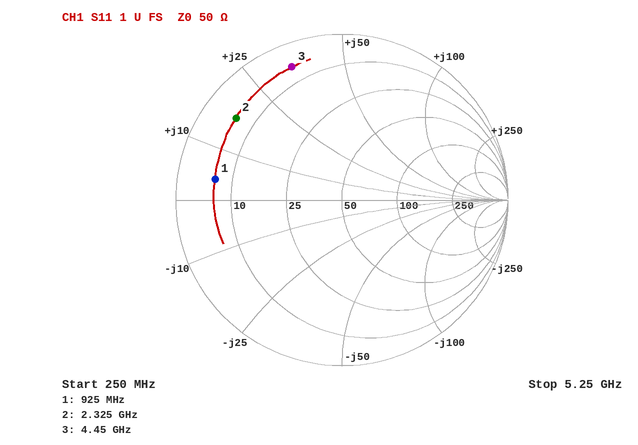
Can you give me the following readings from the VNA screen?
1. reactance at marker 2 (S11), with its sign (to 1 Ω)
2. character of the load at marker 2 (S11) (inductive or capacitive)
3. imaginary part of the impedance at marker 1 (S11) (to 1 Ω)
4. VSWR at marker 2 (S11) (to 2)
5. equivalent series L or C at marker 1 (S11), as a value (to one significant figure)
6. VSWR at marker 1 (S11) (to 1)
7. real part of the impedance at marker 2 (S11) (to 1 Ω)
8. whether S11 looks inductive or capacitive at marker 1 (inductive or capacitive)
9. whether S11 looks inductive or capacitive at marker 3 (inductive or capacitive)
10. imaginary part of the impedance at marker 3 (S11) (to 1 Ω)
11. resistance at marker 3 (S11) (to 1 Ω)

+17 Ω
inductive
+4 Ω
10
700 pH
8
6 Ω
inductive
inductive
+34 Ω
6 Ω
